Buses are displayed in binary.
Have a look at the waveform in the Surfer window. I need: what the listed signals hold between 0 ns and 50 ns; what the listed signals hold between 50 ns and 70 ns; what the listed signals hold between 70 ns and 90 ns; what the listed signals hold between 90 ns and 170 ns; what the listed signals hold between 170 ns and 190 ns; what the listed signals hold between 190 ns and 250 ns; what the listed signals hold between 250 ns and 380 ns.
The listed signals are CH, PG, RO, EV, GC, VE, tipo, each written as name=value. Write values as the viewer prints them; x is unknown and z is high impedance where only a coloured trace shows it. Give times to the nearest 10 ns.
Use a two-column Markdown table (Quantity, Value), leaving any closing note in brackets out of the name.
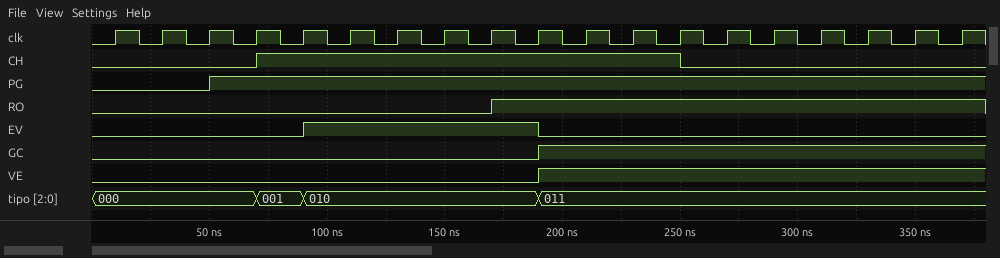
| Quantity | Value |
|---|---|
| what the listed signals hold between 0 ns and 50 ns | CH=0, PG=0, RO=0, EV=0, GC=0, VE=0, tipo=000 |
| what the listed signals hold between 50 ns and 70 ns | CH=0, PG=1, RO=0, EV=0, GC=0, VE=0, tipo=000 |
| what the listed signals hold between 70 ns and 90 ns | CH=1, PG=1, RO=0, EV=0, GC=0, VE=0, tipo=001 |
| what the listed signals hold between 90 ns and 170 ns | CH=1, PG=1, RO=0, EV=1, GC=0, VE=0, tipo=010 |
| what the listed signals hold between 170 ns and 190 ns | CH=1, PG=1, RO=1, EV=1, GC=0, VE=0, tipo=010 |
| what the listed signals hold between 190 ns and 250 ns | CH=1, PG=1, RO=1, EV=0, GC=1, VE=1, tipo=011 |
| what the listed signals hold between 250 ns and 380 ns | CH=0, PG=1, RO=1, EV=0, GC=1, VE=1, tipo=011 |
